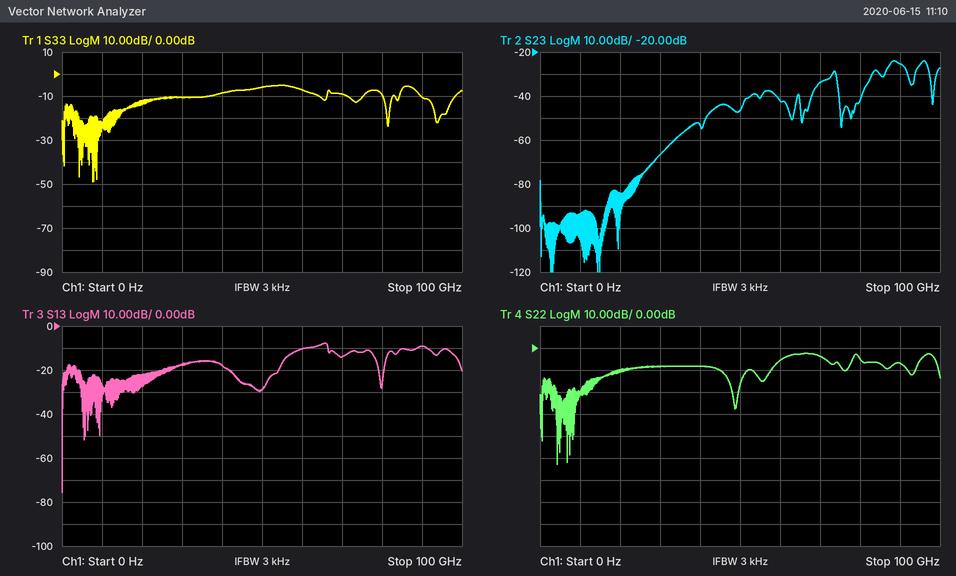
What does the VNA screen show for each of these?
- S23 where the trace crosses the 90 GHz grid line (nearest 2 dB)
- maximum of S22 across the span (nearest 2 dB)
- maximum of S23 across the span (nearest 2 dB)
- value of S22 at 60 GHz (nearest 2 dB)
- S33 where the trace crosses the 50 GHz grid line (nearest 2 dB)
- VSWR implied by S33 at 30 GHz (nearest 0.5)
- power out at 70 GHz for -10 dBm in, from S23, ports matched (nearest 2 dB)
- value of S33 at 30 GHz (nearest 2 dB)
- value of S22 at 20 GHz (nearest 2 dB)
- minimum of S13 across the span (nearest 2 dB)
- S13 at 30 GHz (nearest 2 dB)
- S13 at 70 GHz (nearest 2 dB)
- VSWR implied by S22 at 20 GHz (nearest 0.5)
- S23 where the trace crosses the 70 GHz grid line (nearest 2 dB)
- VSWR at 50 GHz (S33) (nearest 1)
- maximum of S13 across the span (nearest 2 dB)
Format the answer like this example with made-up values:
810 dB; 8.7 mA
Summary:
-26 dB; -2 dB; -24 dB; -6 dB; -6 dB; 2.0; -44 dBm; -10 dB; -10 dB; -76 dB; -18 dB; -14 dB; 2.0; -34 dB; 3; -8 dB
